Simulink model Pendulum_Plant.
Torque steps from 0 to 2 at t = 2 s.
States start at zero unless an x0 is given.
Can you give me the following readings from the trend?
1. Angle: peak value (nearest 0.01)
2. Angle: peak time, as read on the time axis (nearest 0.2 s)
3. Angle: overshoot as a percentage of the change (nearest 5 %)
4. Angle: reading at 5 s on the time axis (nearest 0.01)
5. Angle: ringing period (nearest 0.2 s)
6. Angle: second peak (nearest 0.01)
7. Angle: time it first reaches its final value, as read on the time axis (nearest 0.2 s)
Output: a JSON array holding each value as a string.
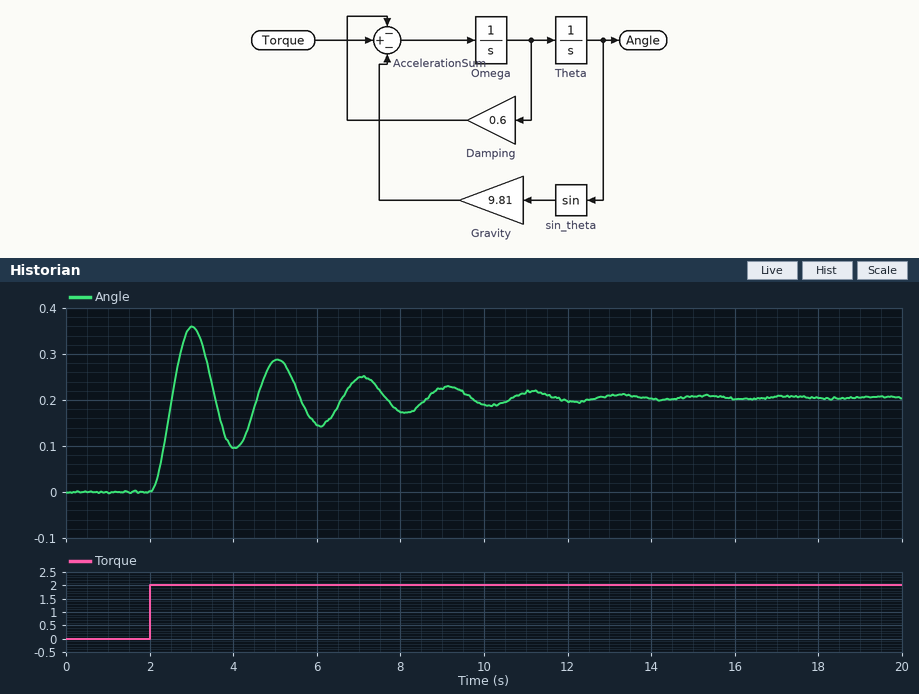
["0.36", "3.0 s", "75 %", "0.29", "2.0 s", "0.29", "2.6 s"]
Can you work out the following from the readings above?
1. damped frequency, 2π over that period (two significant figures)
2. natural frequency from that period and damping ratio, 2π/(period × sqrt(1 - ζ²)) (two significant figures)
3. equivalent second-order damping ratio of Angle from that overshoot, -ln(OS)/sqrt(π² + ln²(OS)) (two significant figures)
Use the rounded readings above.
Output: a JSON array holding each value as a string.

["3.1 rad/s", "3.2 rad/s", "0.091"]
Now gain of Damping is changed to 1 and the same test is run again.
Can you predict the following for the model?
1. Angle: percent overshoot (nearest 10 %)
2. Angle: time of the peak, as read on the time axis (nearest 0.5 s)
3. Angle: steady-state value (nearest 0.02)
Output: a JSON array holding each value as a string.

["60 %", "3.0 s", "0.20"]
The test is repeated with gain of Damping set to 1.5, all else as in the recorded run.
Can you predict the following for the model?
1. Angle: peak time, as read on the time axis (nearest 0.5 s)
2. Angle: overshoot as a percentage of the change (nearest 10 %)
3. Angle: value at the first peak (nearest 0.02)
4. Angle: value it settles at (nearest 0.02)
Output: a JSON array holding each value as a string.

["3.0 s", "50 %", "0.30", "0.20"]
